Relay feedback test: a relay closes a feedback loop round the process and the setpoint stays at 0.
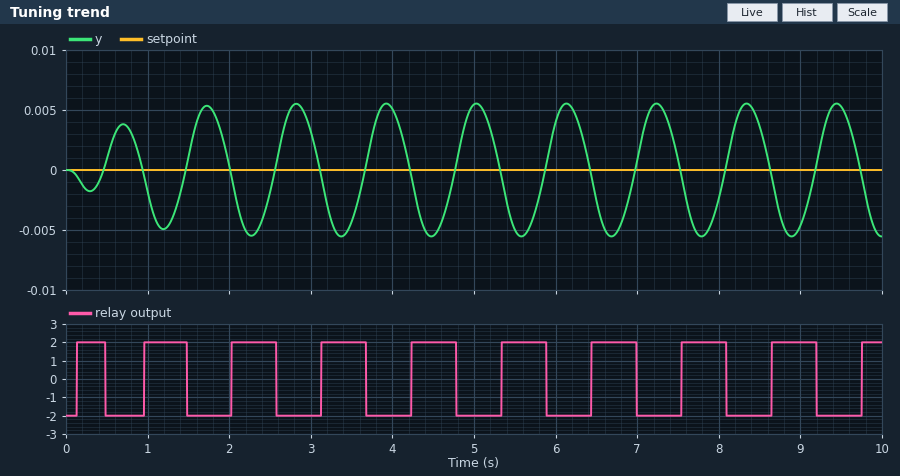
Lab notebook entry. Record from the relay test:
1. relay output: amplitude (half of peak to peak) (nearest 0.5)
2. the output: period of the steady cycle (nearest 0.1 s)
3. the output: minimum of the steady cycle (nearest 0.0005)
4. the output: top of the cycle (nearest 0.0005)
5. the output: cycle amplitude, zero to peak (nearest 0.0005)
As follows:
2.0
1.1 s
-0.0055
0.0055
0.0055
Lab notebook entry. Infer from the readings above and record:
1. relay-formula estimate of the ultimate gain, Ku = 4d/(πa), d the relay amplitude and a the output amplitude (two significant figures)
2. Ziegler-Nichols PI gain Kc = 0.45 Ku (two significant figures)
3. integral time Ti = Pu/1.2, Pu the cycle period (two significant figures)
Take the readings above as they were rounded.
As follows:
460
210
0.92 s
